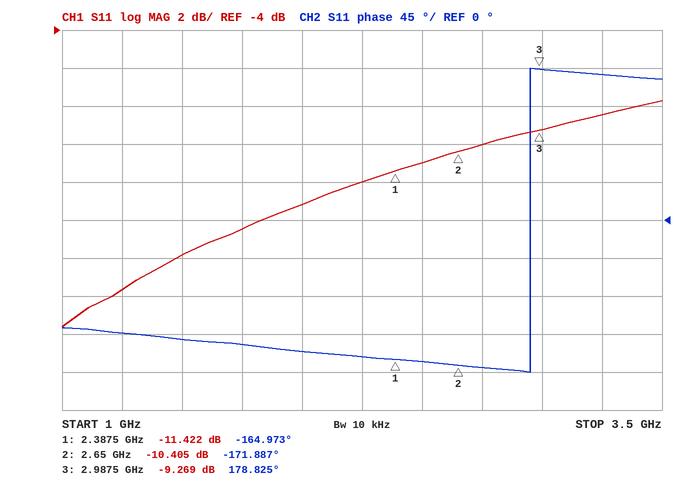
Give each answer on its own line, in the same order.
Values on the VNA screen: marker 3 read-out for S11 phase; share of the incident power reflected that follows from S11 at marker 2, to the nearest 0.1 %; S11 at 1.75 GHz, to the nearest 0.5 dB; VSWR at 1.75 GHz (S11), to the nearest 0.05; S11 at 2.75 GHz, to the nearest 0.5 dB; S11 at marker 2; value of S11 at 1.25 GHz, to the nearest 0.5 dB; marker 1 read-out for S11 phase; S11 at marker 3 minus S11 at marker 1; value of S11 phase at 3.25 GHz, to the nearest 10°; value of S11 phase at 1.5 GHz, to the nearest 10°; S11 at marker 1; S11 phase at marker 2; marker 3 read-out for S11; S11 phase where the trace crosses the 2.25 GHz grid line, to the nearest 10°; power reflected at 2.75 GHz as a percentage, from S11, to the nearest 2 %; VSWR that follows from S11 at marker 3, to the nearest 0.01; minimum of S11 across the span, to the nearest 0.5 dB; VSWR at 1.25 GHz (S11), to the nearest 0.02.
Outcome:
178.825°
9.1 %
-14.5 dB
1.45
-10.0 dB
-10.405 dB
-17.5 dB
-164.973°
2.153 dB
170°
-140°
-11.422 dB
-171.887°
-9.269 dB
-160°
10 %
2.05
-19.5 dB
1.30
